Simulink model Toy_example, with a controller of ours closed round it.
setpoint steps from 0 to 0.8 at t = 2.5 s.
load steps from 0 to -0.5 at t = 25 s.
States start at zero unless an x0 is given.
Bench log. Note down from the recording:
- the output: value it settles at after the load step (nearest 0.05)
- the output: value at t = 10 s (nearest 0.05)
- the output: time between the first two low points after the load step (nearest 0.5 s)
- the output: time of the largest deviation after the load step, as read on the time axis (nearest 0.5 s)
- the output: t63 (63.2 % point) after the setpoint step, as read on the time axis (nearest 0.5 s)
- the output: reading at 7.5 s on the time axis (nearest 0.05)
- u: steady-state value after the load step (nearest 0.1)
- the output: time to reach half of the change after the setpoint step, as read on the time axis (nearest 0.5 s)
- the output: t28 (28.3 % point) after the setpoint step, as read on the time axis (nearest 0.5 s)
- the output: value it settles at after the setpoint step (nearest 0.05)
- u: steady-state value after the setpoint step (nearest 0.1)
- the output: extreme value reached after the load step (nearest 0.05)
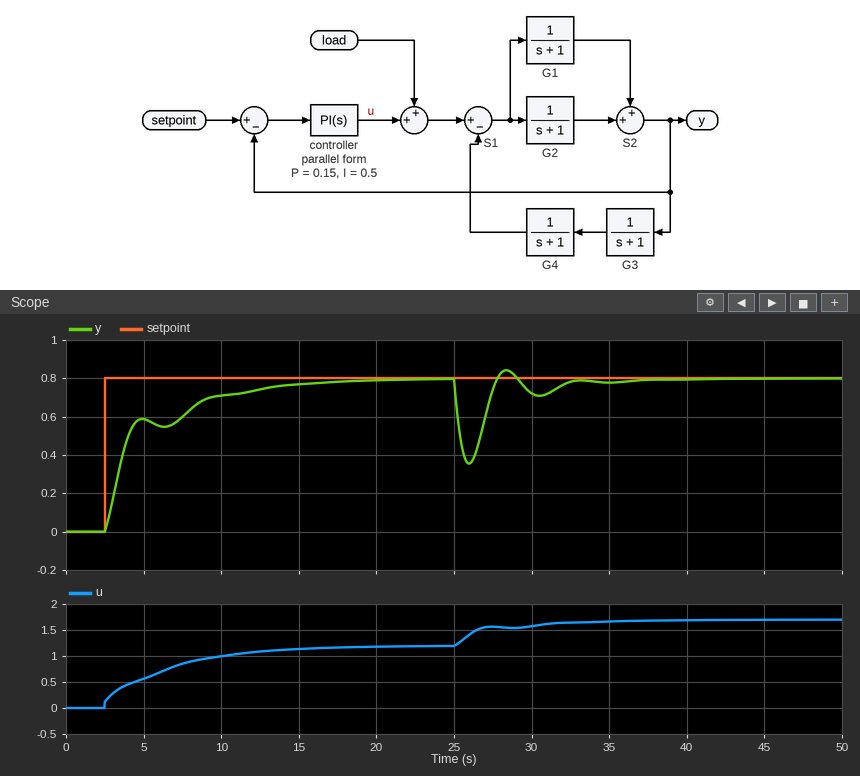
0.80
0.70
4.5 s
26.0 s
4.0 s
0.60
1.7
3.5 s
3.0 s
0.80
1.2
0.35
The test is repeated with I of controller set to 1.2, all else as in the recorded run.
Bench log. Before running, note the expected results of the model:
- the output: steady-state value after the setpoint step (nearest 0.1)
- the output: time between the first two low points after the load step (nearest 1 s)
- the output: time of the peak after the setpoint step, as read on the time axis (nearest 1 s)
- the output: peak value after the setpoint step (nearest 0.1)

0.8
4 s
4 s
0.8
